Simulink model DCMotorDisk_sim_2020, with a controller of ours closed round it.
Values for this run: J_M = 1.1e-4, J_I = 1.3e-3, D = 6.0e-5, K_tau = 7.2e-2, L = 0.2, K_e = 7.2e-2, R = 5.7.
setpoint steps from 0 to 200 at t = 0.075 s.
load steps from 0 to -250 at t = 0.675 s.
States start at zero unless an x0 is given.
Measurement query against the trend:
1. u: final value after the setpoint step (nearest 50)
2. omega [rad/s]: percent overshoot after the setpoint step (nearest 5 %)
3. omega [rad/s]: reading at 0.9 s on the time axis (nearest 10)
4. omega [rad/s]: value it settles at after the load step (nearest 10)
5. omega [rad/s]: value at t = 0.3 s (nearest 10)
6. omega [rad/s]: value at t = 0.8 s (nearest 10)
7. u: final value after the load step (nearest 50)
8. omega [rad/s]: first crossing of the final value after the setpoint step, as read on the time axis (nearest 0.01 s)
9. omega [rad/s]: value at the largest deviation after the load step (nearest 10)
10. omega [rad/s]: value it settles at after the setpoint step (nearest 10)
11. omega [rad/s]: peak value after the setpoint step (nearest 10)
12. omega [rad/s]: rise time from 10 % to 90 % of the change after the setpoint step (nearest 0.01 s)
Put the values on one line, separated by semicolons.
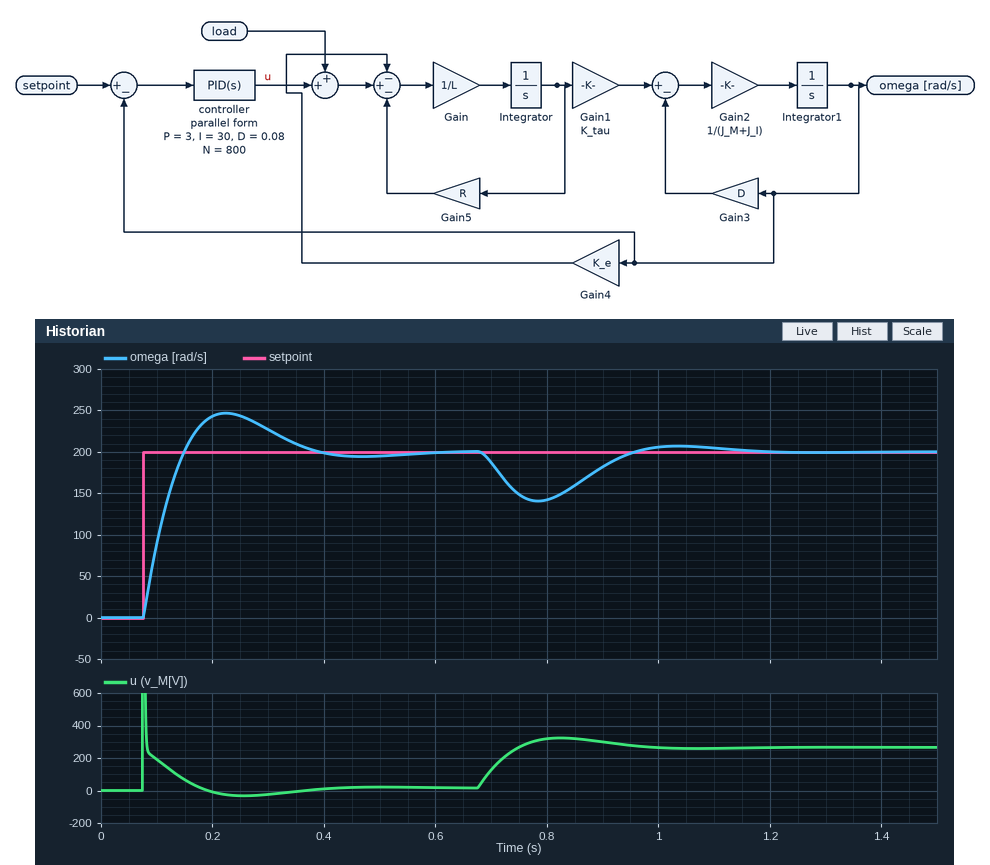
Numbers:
0; 25 %; 180; 200; 230; 140; 250; 0.15 s; 140; 200; 250; 0.06 s
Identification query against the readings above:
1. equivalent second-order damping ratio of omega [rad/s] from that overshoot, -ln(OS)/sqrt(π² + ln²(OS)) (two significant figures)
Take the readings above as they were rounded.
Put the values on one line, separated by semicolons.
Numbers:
0.40
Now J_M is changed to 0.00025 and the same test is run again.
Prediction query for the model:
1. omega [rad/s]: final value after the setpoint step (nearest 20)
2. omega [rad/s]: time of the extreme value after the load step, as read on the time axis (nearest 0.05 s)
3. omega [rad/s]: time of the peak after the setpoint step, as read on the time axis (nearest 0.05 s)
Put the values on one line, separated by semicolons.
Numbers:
200; 0.80 s; 0.25 s
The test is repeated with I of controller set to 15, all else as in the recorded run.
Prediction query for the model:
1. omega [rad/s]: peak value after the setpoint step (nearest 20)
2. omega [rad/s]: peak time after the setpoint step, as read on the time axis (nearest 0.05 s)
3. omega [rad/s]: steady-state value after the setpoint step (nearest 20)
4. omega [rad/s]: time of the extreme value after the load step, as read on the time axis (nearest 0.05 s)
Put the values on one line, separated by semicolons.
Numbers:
220; 0.25 s; 200; 0.80 s
